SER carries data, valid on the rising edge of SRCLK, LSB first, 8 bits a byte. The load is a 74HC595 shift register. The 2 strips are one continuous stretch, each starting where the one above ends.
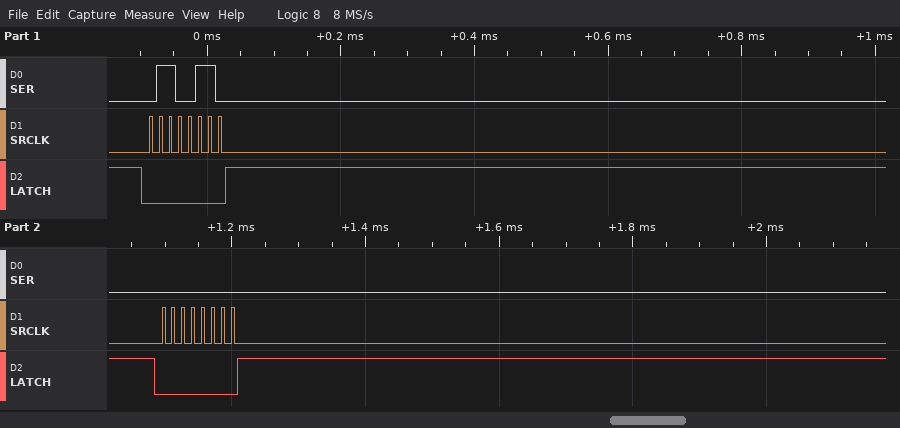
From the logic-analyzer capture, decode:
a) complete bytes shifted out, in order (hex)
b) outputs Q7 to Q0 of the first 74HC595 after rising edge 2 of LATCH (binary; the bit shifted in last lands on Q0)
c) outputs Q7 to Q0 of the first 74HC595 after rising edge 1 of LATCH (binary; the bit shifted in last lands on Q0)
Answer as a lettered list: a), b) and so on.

a) 0x66 0x00
b) 00000000
c) 01100110
